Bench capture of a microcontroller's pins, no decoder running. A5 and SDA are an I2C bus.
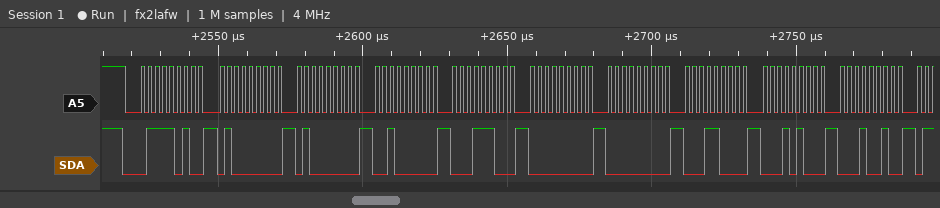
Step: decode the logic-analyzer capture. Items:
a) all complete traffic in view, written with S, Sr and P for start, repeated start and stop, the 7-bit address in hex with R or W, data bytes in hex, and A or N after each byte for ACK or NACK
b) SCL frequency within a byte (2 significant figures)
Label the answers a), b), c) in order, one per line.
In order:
a) S 3DW A 40 A 40 A 20 A 1C A 00 A 00 A 18 A 14 A 12 A
b) 400 kHz
